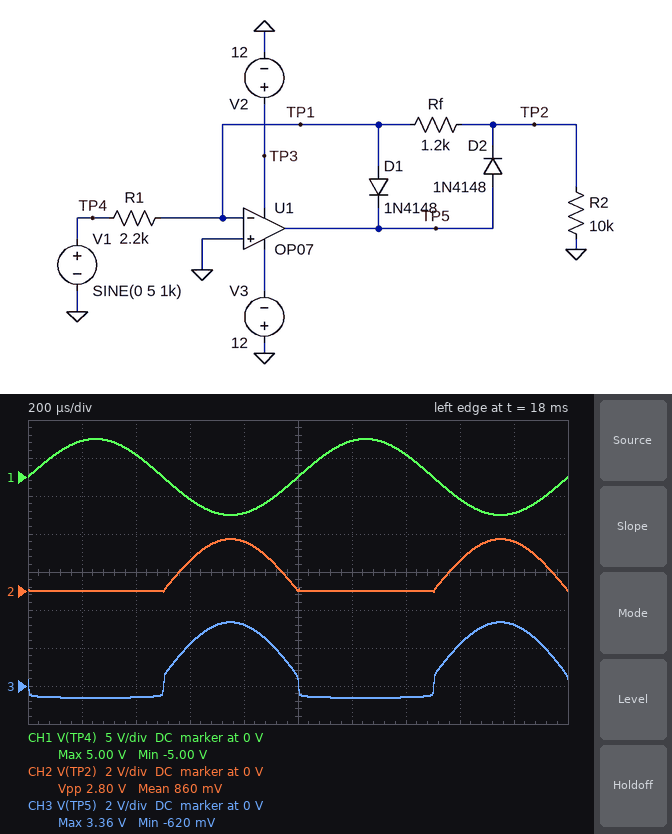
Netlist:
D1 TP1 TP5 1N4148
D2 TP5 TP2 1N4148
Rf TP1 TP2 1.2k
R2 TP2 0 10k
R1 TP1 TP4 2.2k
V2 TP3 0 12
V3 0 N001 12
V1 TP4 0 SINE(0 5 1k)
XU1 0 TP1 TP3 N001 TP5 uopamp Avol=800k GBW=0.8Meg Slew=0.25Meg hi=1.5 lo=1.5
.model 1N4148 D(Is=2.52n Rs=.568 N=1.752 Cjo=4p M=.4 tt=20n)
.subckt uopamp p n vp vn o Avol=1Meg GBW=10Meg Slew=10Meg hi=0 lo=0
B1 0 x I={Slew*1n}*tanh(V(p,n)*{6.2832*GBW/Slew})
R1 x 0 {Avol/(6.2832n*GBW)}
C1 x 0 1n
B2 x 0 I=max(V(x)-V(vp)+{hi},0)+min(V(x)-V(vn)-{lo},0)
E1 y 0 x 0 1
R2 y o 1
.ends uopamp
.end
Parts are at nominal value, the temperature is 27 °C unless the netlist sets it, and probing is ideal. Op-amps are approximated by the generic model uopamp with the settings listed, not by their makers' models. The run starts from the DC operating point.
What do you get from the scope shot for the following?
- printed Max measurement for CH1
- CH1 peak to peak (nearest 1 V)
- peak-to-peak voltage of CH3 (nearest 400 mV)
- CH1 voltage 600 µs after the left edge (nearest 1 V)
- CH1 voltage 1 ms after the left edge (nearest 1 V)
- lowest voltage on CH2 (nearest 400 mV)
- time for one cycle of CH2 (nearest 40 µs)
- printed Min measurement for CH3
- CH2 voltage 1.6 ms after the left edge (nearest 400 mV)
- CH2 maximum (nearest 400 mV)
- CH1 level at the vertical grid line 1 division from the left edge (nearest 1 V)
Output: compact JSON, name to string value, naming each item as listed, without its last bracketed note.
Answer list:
{"printed Max measurement for CH1": "5.00 V", "CH1 peak to peak": "10 V", "peak-to-peak voltage of CH3": "4.0 V", "CH1 voltage 600 µs after the left edge": "-3 V", "CH1 voltage 1 ms after the left edge": "0 V", "lowest voltage on CH2": "0 V", "time for one cycle of CH2": "1.00 ms", "printed Min measurement for CH3": "-620 mV", "CH2 voltage 1.6 ms after the left edge": "1.6 V", "CH2 maximum": "2.8 V", "CH1 level at the vertical grid line 1 division from the left edge": "5 V"}
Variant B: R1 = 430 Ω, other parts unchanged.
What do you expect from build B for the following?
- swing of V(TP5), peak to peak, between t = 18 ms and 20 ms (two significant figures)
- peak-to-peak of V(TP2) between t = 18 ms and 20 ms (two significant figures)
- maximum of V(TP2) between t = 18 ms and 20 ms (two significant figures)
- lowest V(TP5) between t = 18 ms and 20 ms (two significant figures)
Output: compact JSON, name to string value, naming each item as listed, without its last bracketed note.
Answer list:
{"swing of V(TP5), peak to peak, between t = 18 ms and 20 ms": "11 V", "peak-to-peak of V(TP2) between t = 18 ms and 20 ms": "9.9 V", "maximum of V(TP2) between t = 18 ms and 20 ms": "9.8 V", "lowest V(TP5) between t = 18 ms and 20 ms": "-700 mV"}
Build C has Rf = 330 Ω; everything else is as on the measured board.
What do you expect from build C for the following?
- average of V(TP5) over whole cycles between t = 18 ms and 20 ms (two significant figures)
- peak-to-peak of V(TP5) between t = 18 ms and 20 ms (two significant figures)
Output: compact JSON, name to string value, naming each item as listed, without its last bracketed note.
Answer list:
{"average of V(TP5) over whole cycles between t = 18 ms and 20 ms": "240 mV", "peak-to-peak of V(TP5) between t = 18 ms and 20 ms": "2.0 V"}
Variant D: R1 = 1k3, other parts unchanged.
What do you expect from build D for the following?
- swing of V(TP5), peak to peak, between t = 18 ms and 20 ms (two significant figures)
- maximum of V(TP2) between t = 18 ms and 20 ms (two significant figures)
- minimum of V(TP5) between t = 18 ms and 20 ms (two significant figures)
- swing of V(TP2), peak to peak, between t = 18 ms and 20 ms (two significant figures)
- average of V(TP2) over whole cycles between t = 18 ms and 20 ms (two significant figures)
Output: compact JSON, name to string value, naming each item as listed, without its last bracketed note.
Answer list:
{"swing of V(TP5), peak to peak, between t = 18 ms and 20 ms": "5.9 V", "maximum of V(TP2) between t = 18 ms and 20 ms": "4.6 V", "minimum of V(TP5) between t = 18 ms and 20 ms": "-650 mV", "swing of V(TP2), peak to peak, between t = 18 ms and 20 ms": "4.7 V", "average of V(TP2) over whole cycles between t = 18 ms and 20 ms": "1.5 V"}
